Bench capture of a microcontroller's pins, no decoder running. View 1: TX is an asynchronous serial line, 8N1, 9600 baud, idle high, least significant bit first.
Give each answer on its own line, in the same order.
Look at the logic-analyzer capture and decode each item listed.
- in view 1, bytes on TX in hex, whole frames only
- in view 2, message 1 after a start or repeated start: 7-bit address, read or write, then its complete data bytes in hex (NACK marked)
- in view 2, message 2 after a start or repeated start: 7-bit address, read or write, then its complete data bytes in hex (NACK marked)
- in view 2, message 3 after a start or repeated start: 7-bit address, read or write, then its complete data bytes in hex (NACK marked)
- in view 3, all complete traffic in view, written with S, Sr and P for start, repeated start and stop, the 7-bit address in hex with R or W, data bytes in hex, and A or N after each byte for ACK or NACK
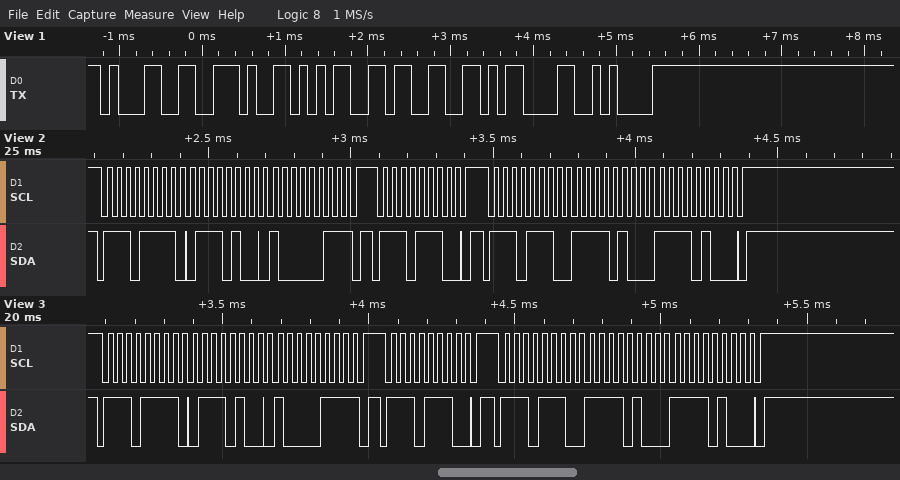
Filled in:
31 2E 35 33 0D 0A
0x77 read: 74 83 NACK
0x77 write
0x77 write: F4 F4
S 77R A 74 A 87 N P S 77W A P S 77W A F4 A F4 A P
